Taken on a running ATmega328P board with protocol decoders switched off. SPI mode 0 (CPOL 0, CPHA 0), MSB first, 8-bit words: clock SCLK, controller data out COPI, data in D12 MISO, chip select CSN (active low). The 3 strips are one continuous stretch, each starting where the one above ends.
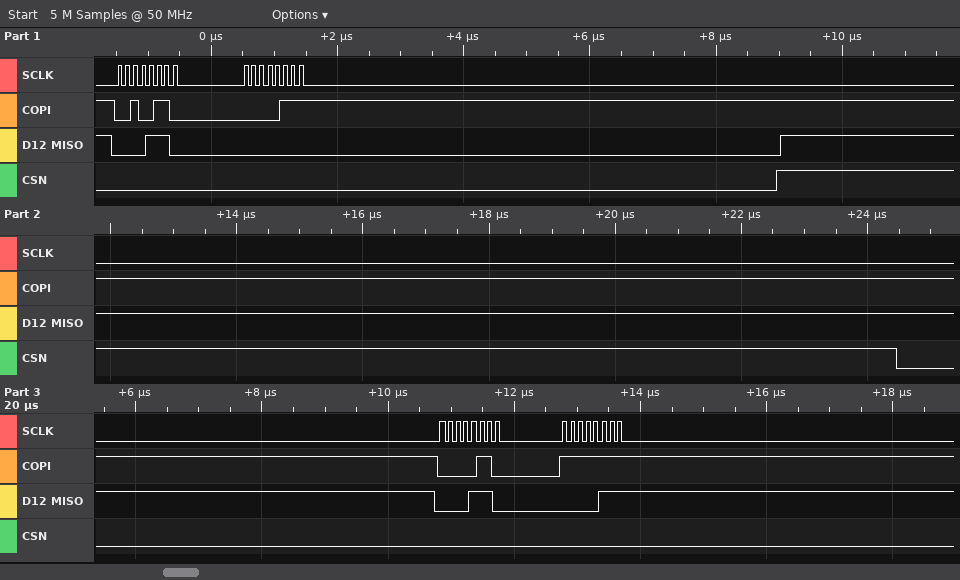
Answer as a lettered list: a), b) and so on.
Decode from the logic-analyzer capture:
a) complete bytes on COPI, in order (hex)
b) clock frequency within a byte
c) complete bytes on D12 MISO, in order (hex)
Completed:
a) 26 07 06 FF
b) 8 MHz
c) 0E 00 0E 07
